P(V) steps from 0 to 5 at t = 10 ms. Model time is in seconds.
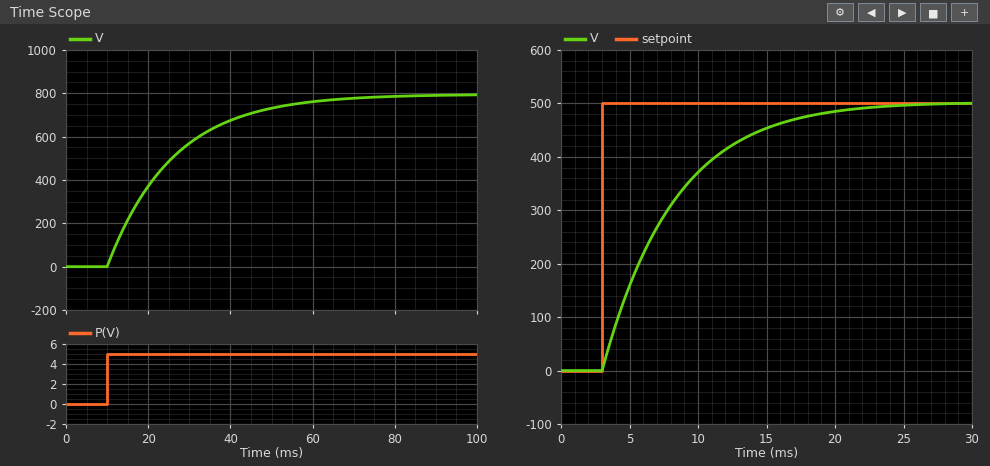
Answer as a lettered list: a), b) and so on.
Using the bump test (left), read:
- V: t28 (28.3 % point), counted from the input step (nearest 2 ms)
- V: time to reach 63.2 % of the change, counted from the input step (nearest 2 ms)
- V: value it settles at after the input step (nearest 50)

a) 6 ms
b) 16 ms
c) 800
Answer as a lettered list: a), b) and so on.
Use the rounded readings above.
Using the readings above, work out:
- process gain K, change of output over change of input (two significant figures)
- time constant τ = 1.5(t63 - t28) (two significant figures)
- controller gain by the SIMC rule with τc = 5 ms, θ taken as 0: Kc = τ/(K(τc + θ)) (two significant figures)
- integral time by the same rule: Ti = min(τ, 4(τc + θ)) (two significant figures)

a) 160
b) 15 ms
c) 0.019
d) 15 ms
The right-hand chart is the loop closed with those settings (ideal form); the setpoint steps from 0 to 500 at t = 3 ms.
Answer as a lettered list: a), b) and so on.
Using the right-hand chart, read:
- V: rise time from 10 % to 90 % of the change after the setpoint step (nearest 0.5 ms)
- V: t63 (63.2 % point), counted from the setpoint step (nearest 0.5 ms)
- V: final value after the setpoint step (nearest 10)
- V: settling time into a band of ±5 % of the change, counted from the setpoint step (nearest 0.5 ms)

a) 11.0 ms
b) 5.0 ms
c) 500
d) 15.0 ms
